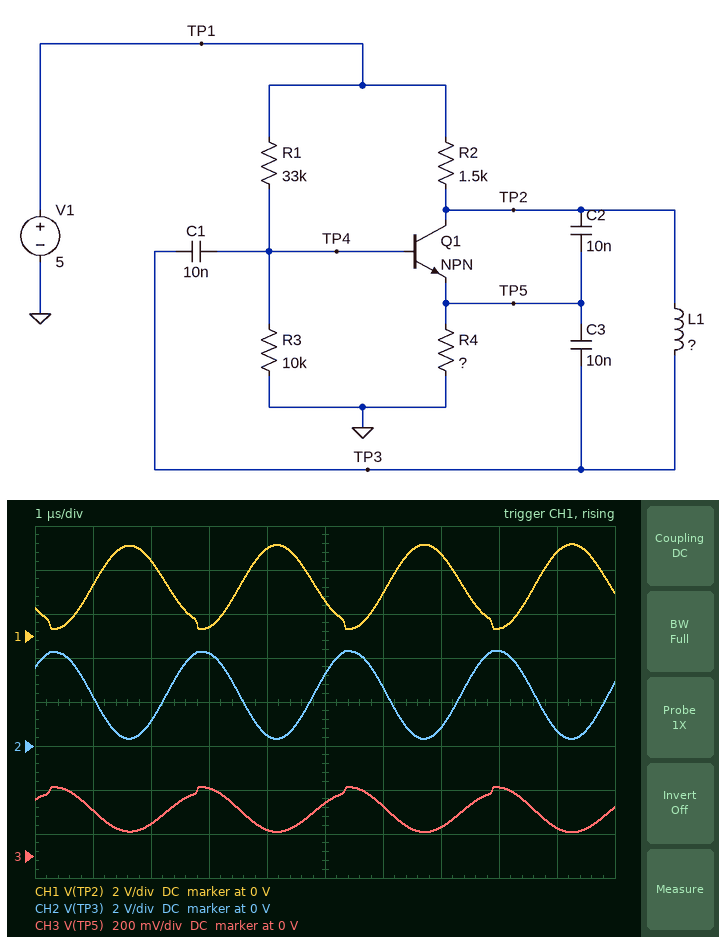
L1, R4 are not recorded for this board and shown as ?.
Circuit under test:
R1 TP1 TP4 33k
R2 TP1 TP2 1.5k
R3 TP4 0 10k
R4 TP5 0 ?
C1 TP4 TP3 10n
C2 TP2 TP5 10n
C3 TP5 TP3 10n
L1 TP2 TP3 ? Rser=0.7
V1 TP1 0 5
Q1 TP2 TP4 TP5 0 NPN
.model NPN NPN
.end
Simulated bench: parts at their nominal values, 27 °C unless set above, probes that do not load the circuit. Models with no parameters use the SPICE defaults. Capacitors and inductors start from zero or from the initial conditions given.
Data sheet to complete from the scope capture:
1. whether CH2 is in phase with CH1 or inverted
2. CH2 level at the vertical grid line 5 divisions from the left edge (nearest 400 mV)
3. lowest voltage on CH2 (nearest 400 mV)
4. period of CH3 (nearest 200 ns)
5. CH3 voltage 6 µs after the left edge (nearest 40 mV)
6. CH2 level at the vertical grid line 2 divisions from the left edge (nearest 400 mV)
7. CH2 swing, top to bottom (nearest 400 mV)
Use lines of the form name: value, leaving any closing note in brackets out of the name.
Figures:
whether CH2 is in phase with CH1 or inverted: inverted
CH2 level at the vertical grid line 5 divisions from the left edge: 3.2 V
lowest voltage on CH2: 400 mV
period of CH3: 2.6 µs
CH3 voltage 6 µs after the left edge: 240 mV
CH2 level at the vertical grid line 2 divisions from the left edge: 1.2 V
CH2 swing, top to bottom: 4.0 V
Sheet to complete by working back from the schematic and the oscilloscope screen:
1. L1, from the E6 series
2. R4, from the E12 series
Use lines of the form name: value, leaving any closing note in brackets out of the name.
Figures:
L1, from the E6 series: 33 µH
R4, from the E12 series: 100 Ω
